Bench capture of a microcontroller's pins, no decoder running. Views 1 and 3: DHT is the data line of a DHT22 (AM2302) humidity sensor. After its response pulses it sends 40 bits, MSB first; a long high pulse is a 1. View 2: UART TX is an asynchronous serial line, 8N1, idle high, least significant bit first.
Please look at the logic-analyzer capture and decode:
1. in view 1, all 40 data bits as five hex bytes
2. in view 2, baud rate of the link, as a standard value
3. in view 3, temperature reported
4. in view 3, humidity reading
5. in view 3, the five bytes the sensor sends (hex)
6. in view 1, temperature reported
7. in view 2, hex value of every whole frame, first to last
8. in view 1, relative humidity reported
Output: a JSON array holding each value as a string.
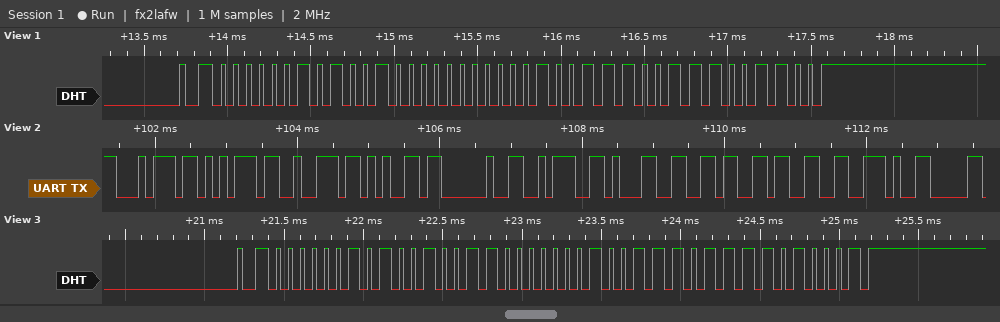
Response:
["02 90 01 39 CC", "9600 baud", "31.5 °C", "65.9 %", "02 93 01 3B D1", "31.3 °C", "74 75 72 65 20 3A 31 36 33 2E", "65.6 %"]
